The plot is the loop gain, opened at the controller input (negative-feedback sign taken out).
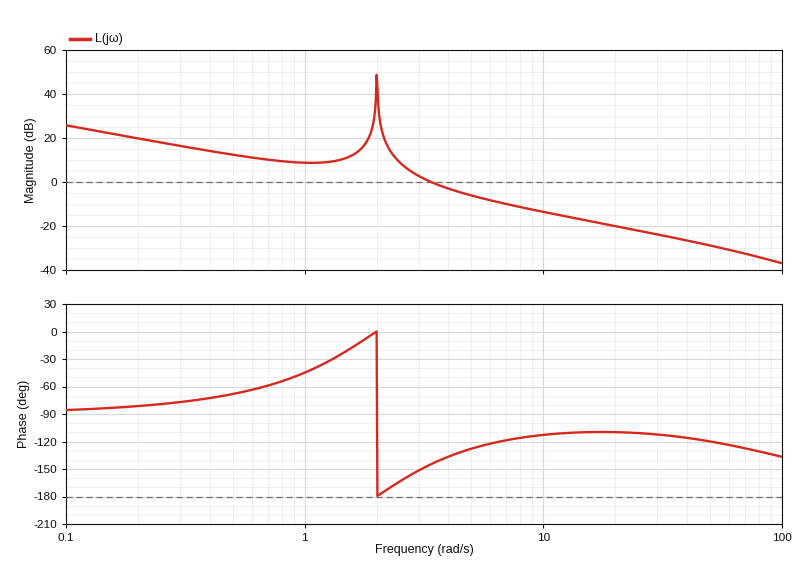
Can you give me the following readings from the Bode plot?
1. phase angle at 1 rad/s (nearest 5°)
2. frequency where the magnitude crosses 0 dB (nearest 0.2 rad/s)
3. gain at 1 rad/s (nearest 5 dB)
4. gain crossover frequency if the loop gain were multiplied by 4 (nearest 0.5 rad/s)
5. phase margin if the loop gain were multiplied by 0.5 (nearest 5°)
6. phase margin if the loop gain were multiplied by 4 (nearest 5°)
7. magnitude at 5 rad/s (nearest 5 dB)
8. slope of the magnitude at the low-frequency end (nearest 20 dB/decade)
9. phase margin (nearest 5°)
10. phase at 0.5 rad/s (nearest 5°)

-45°
3.4 rad/s
10 dB
8.5 rad/s
20°
65°
-5 dB
-20 dB/decade
35°
-70°
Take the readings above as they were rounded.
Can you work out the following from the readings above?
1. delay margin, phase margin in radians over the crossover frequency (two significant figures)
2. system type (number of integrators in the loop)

0.18 s
1
